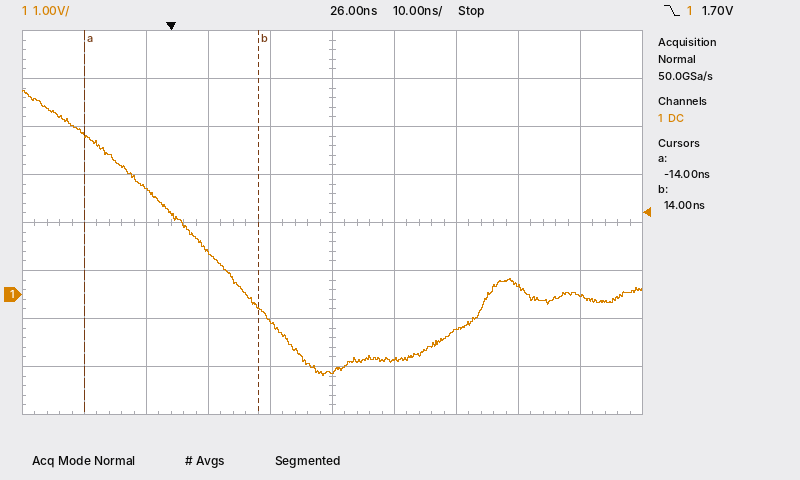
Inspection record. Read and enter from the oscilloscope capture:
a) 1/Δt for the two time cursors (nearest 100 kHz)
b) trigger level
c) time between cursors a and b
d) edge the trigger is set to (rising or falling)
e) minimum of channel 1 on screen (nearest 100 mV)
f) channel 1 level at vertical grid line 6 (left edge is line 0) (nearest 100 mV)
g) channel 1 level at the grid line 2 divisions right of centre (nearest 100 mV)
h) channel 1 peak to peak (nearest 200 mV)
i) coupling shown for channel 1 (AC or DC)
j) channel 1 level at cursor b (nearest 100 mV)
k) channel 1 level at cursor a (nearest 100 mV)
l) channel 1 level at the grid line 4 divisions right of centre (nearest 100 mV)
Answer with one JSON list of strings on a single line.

["35.7 MHz", "1.70 V", "28 ns", "falling", "-1.7 V", "-1.4 V", "-700 mV", "6.0 V", "DC", "-300 mV", "3.3 V", "0.0 V"]
